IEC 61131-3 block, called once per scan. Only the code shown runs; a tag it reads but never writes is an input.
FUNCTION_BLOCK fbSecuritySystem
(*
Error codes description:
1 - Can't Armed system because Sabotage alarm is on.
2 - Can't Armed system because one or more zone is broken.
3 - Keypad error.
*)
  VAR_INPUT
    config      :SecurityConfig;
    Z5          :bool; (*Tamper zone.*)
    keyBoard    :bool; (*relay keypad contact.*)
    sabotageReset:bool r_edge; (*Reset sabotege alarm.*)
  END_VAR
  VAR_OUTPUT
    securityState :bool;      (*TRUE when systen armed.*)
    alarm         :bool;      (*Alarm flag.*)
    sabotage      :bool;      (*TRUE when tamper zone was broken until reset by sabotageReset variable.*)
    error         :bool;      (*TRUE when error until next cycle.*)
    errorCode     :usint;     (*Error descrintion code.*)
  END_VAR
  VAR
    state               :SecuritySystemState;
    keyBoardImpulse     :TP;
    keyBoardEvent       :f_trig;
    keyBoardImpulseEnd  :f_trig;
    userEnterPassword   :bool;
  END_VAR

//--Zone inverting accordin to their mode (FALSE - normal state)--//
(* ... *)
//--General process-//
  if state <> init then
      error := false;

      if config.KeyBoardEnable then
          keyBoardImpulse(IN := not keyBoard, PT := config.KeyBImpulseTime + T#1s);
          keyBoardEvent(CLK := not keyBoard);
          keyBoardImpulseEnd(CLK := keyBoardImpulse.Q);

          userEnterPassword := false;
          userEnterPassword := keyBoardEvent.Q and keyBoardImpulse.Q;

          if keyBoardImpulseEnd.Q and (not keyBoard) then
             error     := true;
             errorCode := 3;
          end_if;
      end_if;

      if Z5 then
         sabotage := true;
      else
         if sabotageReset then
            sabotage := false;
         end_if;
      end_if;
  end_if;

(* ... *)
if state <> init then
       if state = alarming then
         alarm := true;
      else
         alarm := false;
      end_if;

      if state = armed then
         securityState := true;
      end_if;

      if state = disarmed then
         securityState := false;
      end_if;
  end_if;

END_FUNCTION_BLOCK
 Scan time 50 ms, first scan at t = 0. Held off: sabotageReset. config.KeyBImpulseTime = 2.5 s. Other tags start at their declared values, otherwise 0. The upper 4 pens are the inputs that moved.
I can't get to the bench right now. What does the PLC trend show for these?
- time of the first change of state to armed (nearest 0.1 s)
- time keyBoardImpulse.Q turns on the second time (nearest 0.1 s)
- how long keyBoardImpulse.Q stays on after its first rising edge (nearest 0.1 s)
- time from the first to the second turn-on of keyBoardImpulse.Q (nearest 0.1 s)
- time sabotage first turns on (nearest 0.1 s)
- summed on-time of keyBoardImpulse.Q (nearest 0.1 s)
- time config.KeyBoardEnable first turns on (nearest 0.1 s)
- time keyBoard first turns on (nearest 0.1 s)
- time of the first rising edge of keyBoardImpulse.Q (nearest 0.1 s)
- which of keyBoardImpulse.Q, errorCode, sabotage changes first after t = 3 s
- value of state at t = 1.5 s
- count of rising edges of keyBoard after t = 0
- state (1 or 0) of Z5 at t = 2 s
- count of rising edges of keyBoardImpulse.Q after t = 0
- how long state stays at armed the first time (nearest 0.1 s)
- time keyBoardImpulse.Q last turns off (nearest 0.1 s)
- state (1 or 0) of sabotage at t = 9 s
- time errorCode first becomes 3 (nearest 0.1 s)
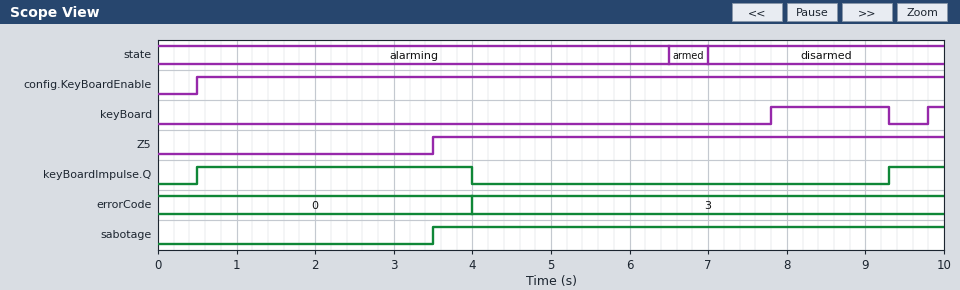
6.5 s
9.3 s
3.5 s
8.8 s
3.5 s
4.2 s
0.5 s
7.8 s
0.5 s
sabotage
alarming
2
0
2
0.5 s
4.0 s
1
4.0 s
